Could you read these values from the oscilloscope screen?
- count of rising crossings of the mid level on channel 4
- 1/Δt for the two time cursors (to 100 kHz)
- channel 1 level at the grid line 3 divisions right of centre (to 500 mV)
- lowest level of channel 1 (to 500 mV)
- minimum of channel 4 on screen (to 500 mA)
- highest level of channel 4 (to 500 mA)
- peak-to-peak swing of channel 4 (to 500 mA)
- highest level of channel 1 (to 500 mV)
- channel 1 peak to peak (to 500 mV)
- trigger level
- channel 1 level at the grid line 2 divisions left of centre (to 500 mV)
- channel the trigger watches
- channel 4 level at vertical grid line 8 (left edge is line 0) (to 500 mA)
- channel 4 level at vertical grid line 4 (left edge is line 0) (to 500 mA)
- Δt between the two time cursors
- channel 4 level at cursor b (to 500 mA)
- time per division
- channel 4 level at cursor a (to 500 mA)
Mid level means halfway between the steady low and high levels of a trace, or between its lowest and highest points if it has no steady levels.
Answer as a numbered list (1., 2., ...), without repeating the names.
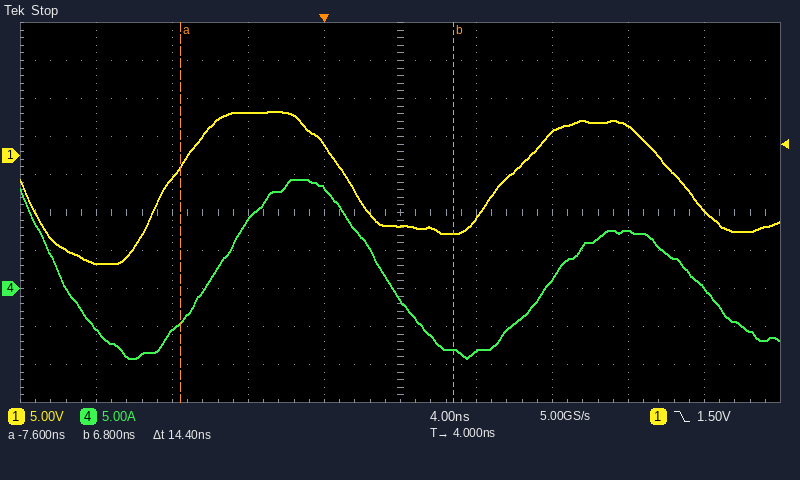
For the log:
1. 2
2. 69.4 MHz
3. 4.0 V
4. -14.0 V
5. -9.0 A
6. 14.5 A
7. 23.5 A
8. 6.0 V
9. 20.0 V
10. 1.50 V
11. 5.5 V
12. channel 1
13. 7.5 A
14. 13.0 A
15. 14.4 ns
16. -8.0 A
17. 4 ns
18. -4.5 A
